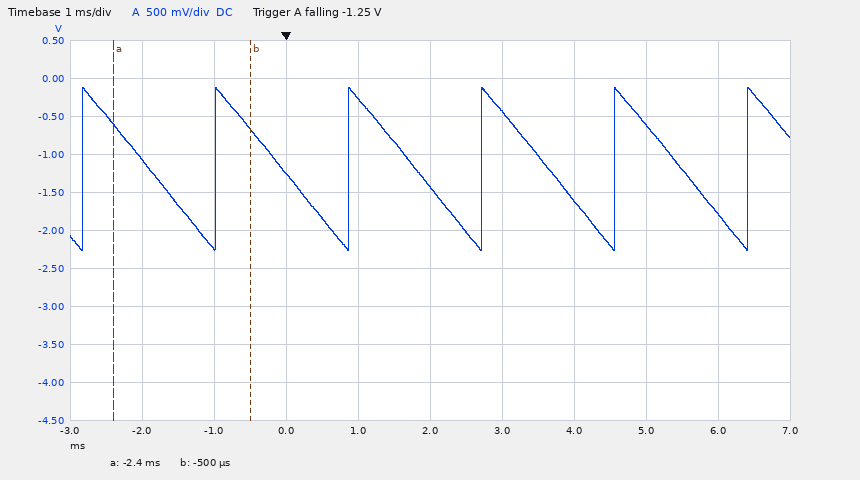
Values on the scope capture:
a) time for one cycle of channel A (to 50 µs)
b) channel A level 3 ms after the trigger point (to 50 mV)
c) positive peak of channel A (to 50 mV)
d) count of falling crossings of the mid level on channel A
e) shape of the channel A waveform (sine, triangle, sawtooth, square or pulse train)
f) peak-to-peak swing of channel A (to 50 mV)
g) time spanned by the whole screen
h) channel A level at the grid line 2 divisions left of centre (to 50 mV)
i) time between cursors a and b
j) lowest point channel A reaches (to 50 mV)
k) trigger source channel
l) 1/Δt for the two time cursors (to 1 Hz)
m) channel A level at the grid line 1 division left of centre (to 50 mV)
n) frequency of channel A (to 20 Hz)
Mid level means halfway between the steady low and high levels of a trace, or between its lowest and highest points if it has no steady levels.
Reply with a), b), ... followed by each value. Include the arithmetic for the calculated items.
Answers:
a) 1.85 ms
b) -450 mV
c) -100 mV
d) 5
e) sawtooth
f) -100 mV − (-2.25 V) = 2.15 V
g) 10 ms
h) -1.25 V
i) -500 µs − (-2.4 ms) = 1.9 ms
j) -2.25 V
k) channel A
l) 1 / 1.9 ms ≈ 526 Hz
m) -250 mV
n) 1 / 1.85 ms ≈ 541 Hz, so 540 Hz to the nearest 20 Hz
